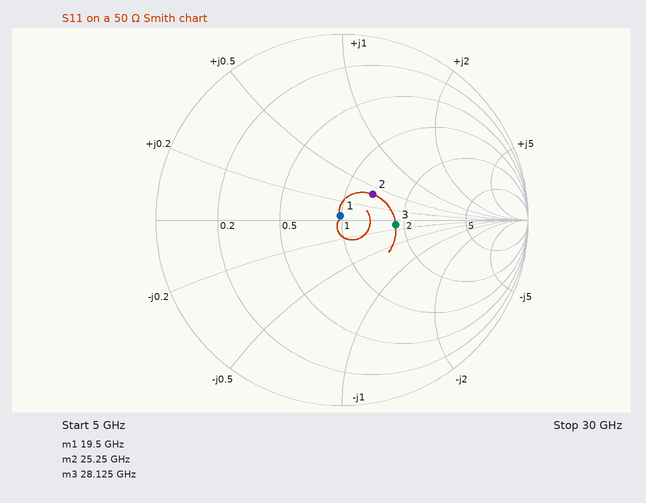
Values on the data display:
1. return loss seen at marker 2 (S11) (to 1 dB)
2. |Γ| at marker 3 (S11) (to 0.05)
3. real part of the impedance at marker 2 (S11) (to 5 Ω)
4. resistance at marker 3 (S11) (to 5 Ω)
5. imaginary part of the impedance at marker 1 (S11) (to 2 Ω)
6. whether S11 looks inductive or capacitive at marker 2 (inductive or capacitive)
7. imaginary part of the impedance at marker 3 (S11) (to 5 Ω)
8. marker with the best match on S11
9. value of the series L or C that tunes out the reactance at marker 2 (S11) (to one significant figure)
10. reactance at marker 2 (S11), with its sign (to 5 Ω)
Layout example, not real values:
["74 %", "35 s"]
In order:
["13 dB", "0.30", "65 Ω", "90 Ω", "+2 Ω", "inductive", "-5 Ω", "marker 1", "300 fF", "+20 Ω"]
